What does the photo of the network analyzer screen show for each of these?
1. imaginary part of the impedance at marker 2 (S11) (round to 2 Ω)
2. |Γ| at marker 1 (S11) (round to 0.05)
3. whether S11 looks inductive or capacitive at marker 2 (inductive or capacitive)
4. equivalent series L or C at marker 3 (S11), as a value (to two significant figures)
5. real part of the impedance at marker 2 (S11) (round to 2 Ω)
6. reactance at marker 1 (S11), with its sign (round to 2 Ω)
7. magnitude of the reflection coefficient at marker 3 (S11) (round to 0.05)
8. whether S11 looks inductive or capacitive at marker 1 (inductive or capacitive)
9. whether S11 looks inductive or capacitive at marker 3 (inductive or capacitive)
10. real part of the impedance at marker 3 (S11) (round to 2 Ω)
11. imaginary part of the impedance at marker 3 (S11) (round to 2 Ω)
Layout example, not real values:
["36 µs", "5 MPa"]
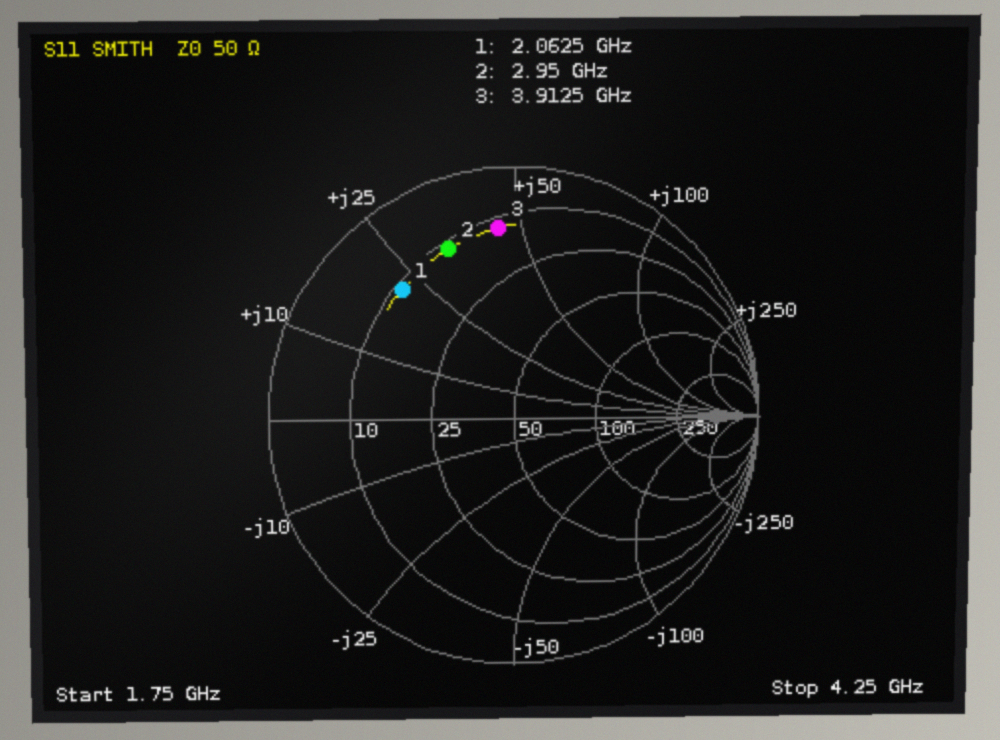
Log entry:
["+32 Ω", "0.70", "inductive", "1.8 nH", "12 Ω", "+22 Ω", "0.75", "inductive", "inductive", "12 Ω", "+44 Ω"]
